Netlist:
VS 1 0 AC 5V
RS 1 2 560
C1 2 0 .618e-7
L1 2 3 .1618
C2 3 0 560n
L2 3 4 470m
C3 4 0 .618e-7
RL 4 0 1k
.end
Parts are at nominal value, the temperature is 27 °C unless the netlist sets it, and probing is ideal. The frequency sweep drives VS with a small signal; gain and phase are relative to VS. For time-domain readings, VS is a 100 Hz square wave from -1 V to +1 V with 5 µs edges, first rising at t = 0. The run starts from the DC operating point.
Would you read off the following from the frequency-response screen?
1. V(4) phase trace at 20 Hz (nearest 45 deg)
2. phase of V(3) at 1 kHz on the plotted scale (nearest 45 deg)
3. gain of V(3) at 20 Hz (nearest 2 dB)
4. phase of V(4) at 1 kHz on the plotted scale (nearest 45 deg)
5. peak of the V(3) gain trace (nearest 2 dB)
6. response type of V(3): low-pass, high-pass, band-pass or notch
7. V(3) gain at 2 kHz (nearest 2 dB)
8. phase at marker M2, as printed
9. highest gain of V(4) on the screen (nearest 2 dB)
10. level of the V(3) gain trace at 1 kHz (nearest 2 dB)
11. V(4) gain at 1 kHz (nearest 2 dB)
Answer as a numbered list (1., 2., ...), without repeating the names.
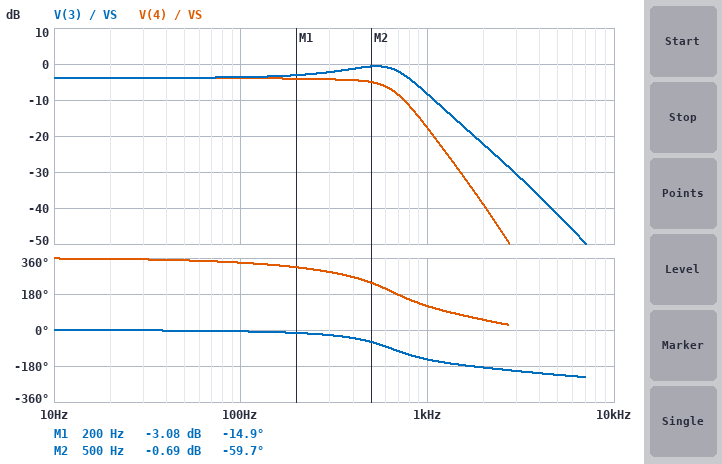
1. 360 deg
2. -135 deg
3. -4 dB
4. 135 deg
5. 0 dB
6. low-pass
7. -22 dB
8. -59.7 deg
9. -4 dB
10. -8 dB
11. -18 dB
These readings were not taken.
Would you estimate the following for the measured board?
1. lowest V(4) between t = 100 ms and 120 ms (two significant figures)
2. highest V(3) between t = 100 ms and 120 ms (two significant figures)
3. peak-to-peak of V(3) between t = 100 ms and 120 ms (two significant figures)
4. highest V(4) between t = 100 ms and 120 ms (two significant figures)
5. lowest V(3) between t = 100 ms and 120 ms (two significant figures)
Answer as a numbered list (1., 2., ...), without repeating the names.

1. -730 mV
2. 1.0 V
3. 2.1 V
4. 730 mV
5. -1.0 V
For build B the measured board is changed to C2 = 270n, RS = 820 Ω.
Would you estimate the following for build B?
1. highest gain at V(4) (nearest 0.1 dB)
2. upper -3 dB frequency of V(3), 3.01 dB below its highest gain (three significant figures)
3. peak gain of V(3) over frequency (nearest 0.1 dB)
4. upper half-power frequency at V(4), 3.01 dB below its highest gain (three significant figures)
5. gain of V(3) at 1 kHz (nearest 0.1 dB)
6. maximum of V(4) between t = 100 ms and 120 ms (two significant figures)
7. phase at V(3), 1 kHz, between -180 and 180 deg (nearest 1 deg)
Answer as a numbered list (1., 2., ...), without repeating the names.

1. -5.2 dB
2. 1.17 kHz
3. -0.3 dB
4. 836 Hz
5. -1.2 dB
6. 590 mV
7. -106 deg
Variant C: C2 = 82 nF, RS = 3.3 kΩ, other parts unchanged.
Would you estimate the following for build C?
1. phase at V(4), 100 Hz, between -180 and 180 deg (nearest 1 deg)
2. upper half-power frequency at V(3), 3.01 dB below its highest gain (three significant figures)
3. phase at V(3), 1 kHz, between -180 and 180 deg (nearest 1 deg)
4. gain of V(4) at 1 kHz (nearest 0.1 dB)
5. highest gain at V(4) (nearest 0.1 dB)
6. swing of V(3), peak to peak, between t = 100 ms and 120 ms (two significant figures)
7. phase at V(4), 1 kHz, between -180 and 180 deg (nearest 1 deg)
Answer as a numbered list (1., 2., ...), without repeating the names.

1. -11 deg
2. 2.29 kHz
3. -59 deg
4. -15.6 dB
5. -11.2 dB
6. 1.5 V
7. -152 deg
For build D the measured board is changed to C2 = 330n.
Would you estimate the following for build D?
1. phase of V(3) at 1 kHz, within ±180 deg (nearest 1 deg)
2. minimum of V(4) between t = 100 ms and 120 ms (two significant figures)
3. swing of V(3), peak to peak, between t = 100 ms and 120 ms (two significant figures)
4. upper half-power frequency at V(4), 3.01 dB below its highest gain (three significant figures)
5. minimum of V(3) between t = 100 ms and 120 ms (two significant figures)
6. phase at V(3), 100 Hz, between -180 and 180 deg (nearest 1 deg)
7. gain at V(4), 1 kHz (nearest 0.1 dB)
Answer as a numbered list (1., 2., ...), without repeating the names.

1. -128 deg
2. -700 mV
3. 2.4 V
4. 848 Hz
5. -1.2 V
6. -4 deg
7. -10.8 dB
